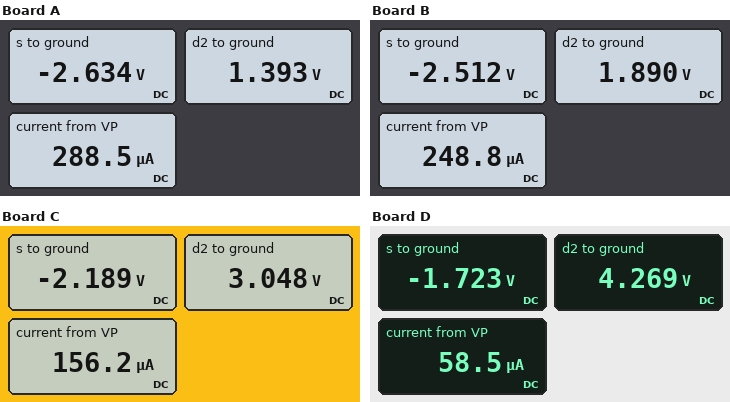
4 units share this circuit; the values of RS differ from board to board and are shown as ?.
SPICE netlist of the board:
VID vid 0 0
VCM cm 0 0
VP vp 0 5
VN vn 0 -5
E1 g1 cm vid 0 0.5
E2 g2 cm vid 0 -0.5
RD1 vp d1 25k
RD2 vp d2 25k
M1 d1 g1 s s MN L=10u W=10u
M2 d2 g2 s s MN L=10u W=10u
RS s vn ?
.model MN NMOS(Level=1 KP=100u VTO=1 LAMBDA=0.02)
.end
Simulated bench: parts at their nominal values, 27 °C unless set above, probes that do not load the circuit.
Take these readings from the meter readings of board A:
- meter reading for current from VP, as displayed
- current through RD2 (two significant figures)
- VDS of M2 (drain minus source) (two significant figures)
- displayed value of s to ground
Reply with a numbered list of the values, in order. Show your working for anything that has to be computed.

1. 288.5 µA
2. (5 V - 1.393 V) / 25 kΩ = 140 µA
3. 1.393 V - (-2.634 V) = 4.0 V
4. -2.634 V
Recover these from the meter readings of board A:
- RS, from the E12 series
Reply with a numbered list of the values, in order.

1. 8.2 kΩ
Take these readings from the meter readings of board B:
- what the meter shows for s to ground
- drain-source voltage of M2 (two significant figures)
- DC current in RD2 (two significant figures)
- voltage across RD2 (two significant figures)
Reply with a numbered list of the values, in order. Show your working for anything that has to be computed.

1. -2.512 V
2. 1.89 V - (-2.512 V) = 4.4 V
3. (5 V - 1.89 V) / 25 kΩ = 120 µA
4. 5 V - 1.89 V = 3.1 V
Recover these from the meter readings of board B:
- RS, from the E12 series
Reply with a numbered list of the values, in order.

1. 10 kΩ
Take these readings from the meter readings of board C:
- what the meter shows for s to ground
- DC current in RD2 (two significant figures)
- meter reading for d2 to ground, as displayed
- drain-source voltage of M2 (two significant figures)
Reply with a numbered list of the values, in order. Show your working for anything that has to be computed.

1. -2.189 V
2. (5 V - 3.048 V) / 25 kΩ = 78 µA
3. 3.048 V
4. 3.048 V - (-2.189 V) = 5.2 V
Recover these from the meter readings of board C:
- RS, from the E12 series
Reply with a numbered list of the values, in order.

1. 18 kΩ
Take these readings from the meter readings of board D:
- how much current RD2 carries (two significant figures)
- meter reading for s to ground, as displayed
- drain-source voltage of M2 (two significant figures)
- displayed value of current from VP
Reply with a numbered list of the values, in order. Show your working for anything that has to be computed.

1. (5 V - 4.269 V) / 25 kΩ = 29 µA
2. -1.723 V
3. 4.269 V - (-1.723 V) = 6.0 V
4. 58.5 µA
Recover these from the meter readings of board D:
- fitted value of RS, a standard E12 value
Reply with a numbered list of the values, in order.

1. 56 kΩ
